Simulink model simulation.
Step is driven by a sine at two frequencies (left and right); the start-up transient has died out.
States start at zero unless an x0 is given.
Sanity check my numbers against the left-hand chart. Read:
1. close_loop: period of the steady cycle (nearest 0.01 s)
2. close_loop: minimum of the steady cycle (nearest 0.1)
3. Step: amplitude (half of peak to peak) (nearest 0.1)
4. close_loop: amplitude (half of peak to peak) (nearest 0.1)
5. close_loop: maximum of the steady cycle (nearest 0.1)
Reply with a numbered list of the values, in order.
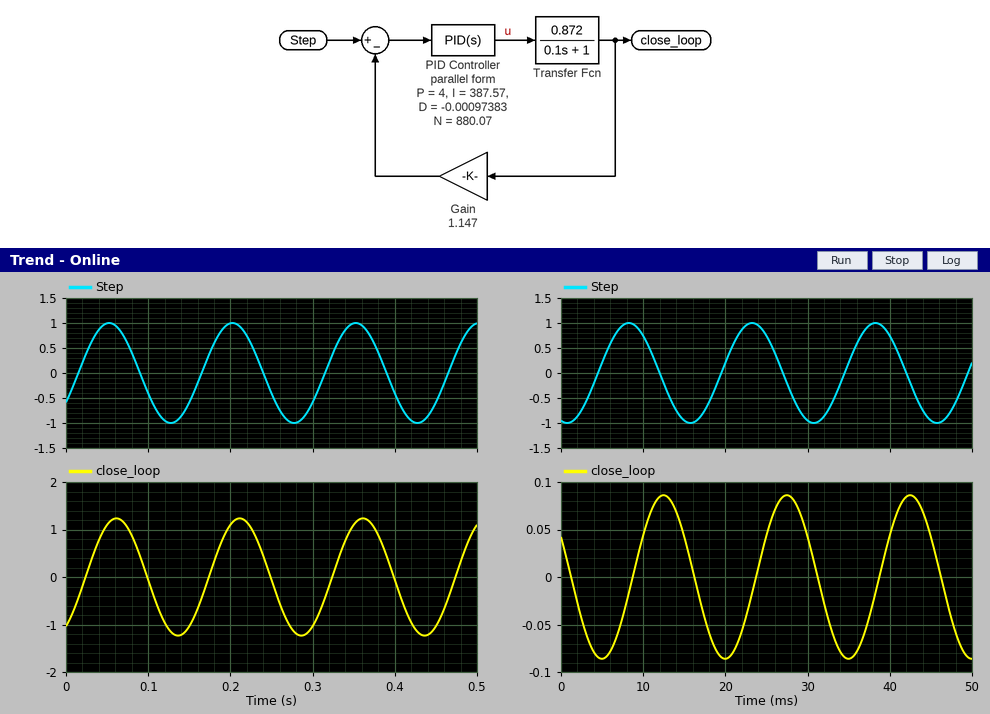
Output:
1. 0.15 s
2. -1.2
3. 1.0
4. 1.2
5. 1.2
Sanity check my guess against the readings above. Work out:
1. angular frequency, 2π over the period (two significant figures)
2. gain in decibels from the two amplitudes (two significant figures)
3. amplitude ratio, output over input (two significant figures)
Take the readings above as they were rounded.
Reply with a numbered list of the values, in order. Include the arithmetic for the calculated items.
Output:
1. 2π / 0.15 = 42 rad/s
2. 20 log10(1.2 / 1) = 1.6 dB
3. 1.2 / 1 = 1.2
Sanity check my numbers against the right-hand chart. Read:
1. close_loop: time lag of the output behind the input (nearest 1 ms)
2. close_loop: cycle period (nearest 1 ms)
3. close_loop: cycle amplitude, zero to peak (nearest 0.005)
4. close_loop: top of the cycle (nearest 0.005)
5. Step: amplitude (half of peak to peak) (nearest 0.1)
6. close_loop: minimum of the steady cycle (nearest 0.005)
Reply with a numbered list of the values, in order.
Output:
1. 4 ms
2. 15 ms
3. 0.085
4. 0.085
5. 1.0
6. -0.085
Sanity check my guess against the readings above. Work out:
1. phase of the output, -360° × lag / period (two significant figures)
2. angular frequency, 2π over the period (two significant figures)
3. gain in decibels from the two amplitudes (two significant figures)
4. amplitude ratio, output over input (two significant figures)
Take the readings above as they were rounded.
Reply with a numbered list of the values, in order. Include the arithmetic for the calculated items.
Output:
1. -360 × 4 / 15 = -96°
2. 2π / 15 = 0.42 rad/ms
3. 20 log10(0.085 / 1) = -21 dB
4. 0.085 / 1 = 0.085
